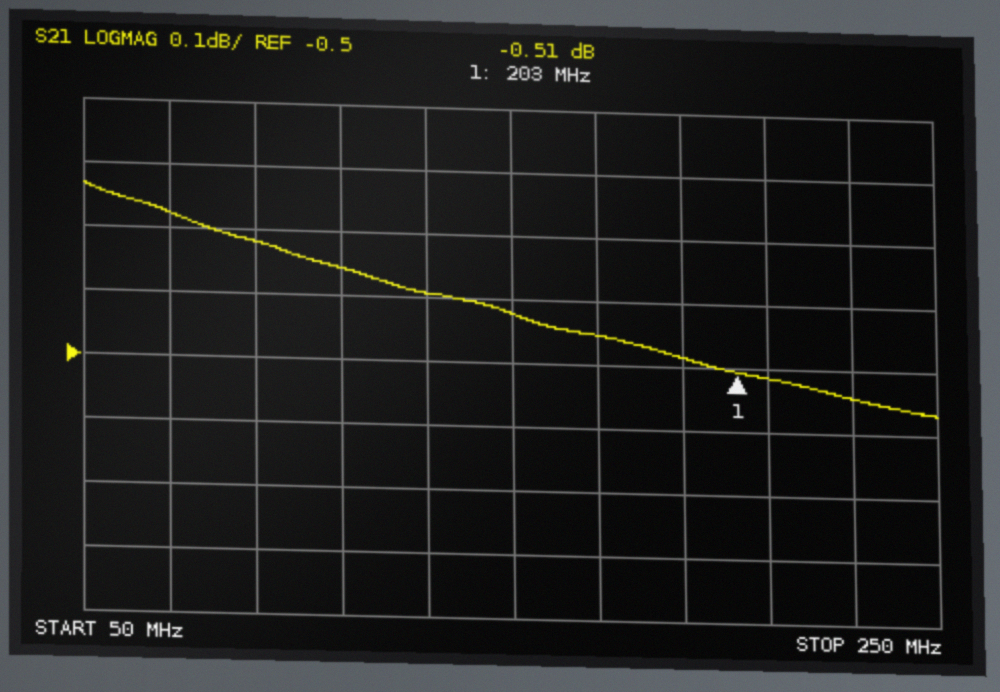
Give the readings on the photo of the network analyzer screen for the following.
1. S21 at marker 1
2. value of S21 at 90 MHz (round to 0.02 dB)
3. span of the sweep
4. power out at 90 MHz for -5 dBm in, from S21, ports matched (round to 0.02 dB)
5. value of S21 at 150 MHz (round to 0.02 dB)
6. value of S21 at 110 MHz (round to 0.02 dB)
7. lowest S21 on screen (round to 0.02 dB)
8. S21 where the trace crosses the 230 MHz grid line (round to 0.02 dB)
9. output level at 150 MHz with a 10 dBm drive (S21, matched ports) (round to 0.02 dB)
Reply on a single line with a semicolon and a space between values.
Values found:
-0.51 dB; -0.32 dB; 200 MHz; -5.32 dBm; -0.42 dB; -0.36 dB; -0.56 dB; -0.54 dB; 9.58 dBm
